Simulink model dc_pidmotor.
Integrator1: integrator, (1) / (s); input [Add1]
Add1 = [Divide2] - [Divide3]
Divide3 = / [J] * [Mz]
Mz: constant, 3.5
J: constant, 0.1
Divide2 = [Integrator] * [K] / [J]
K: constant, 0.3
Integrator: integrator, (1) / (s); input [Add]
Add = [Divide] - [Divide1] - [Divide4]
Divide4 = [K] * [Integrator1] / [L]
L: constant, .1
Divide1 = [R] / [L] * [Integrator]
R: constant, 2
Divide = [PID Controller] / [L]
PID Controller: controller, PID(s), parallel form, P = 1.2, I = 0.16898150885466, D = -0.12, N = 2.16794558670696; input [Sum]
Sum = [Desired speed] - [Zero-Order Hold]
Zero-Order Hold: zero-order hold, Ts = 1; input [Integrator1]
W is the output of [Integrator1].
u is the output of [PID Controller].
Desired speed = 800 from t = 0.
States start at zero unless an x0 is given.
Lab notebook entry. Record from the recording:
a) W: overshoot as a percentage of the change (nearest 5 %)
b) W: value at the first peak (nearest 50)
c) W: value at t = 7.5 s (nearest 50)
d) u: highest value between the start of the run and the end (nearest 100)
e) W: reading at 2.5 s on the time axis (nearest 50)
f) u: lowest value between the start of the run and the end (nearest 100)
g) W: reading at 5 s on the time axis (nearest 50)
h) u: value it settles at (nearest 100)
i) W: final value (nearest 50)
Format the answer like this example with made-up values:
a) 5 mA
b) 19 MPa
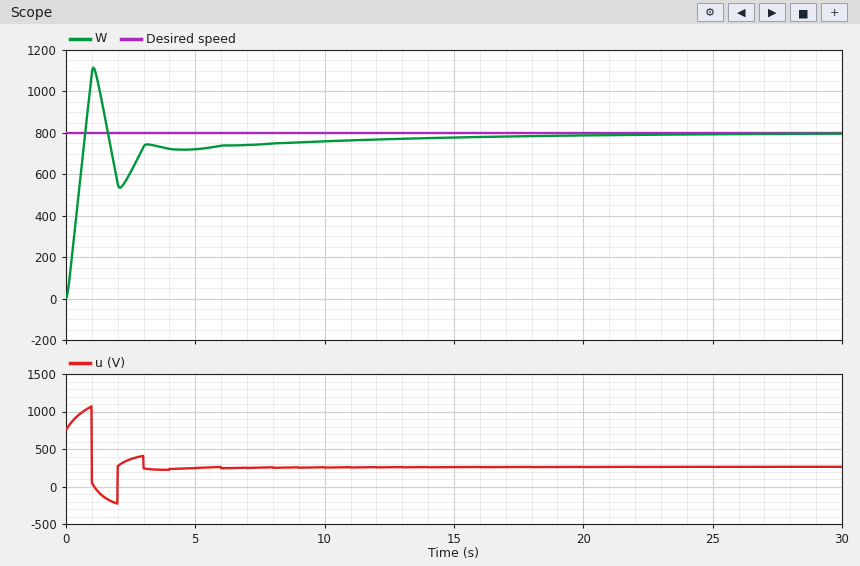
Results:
a) 40 %
b) 1100
c) 750
d) 1100
e) 600
f) -200
g) 700
h) 300
i) 800
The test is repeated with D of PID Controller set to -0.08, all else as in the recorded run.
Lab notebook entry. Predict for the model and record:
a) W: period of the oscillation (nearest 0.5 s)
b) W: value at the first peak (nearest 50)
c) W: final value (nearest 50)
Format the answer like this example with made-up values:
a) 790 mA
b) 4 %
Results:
a) 2.0 s
b) 1150
c) 800
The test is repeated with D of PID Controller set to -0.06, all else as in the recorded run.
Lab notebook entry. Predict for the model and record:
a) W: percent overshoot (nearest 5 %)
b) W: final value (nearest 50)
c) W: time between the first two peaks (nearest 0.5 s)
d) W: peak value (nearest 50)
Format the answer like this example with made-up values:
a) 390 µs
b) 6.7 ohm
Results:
a) 45 %
b) 800
c) 2.0 s
d) 1150
